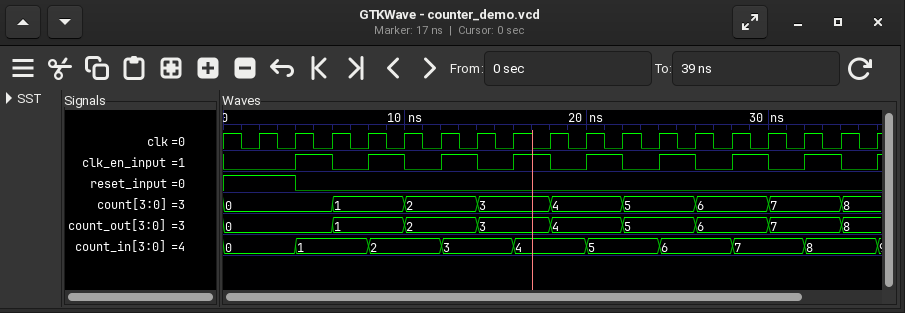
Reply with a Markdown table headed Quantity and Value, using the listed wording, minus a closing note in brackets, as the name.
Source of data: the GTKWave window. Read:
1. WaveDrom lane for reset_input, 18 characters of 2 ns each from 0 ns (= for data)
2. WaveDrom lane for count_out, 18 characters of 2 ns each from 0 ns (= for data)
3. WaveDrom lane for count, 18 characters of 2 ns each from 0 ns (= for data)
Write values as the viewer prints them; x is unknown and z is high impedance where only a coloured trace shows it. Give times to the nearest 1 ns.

| Quantity | Value |
|---|---|
| WaveDrom lane for reset_input, 18 characters of 2 ns each from 0 ns | {name: 'reset_input', wave: '1.0...............'} |
| WaveDrom lane for count_out, 18 characters of 2 ns each from 0 ns | {name: 'count_out', wave: '=..=.=.=.=.=.=.=.=', data: '0 1 2 3 4 5 6 7 8'} |
| WaveDrom lane for count, 18 characters of 2 ns each from 0 ns | {name: 'count', wave: '=..=.=.=.=.=.=.=.=', data: '0 1 2 3 4 5 6 7 8'} |
